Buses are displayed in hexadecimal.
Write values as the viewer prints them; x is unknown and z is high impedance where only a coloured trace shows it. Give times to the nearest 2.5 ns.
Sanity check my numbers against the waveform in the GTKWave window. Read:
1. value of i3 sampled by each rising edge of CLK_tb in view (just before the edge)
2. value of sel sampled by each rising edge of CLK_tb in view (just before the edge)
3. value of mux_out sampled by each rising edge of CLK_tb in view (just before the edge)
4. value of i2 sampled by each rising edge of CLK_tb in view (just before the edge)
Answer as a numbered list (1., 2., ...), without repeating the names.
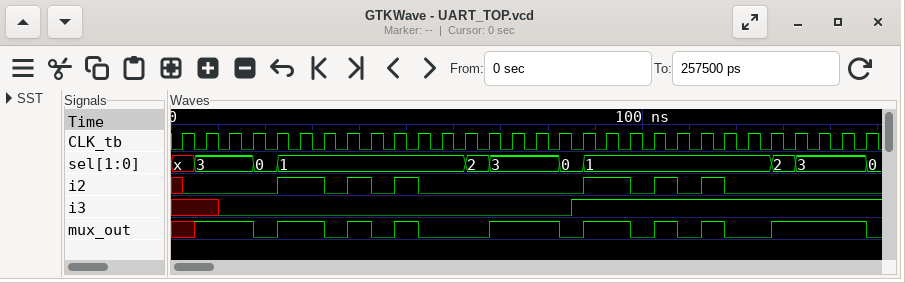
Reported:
1. x x 0 0 0 0 0 0 0 0 0 0 0 0 0 0 0 1 1 1 1 1 1 1 1 1 1 1 1 1
2. x, 3, 3, 3, 0, 1, 1, 1, 1, 1, 1, 1, 1, 2, 3, 3, 3, 0, 1, 1, 1, 1, 1, 1, 1, 1, 2, 3, 3, 3
3. x 1 1 1 0 1 1 0 1 0 1 0 0 0 1 1 1 0 1 1 0 1 0 1 0 0 1 1 1 1
4. x 0 0 0 0 1 1 0 1 0 1 0 0 0 0 0 0 0 1 1 0 1 0 1 0 0 0 0 0 0
